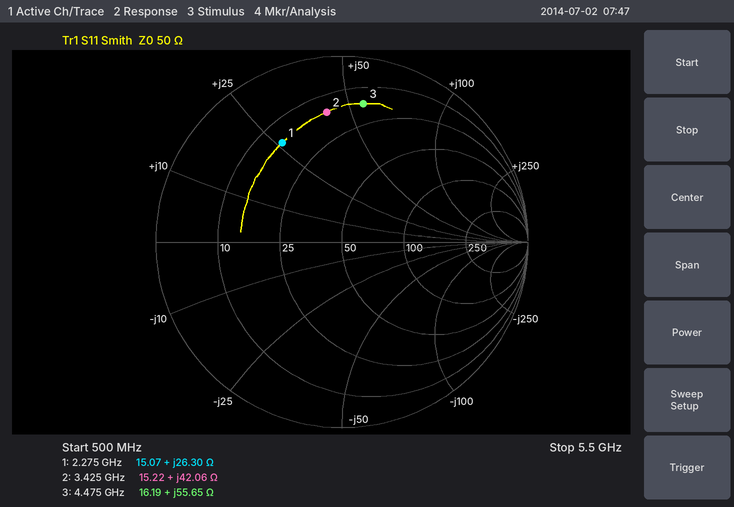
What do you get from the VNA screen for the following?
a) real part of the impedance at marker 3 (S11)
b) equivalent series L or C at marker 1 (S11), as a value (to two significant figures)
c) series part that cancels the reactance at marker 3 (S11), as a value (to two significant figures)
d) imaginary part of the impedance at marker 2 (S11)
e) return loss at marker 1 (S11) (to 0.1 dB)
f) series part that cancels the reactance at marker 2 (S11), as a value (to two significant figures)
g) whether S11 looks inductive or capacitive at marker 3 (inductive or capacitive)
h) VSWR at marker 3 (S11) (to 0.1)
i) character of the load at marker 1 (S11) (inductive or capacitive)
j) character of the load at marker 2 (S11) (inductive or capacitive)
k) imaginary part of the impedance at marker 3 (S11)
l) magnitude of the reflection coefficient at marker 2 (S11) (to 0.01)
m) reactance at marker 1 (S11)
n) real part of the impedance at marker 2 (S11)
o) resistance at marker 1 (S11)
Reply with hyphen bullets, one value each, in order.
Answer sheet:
- 16.19 Ω
- 1.8 nH
- 640 fF
- +42.06 Ω
- 4.1 dB
- 1.1 pF
- inductive
- 7.1
- inductive
- inductive
- +55.65 Ω
- 0.70
- +26.30 Ω
- 15.22 Ω
- 15.07 Ω
